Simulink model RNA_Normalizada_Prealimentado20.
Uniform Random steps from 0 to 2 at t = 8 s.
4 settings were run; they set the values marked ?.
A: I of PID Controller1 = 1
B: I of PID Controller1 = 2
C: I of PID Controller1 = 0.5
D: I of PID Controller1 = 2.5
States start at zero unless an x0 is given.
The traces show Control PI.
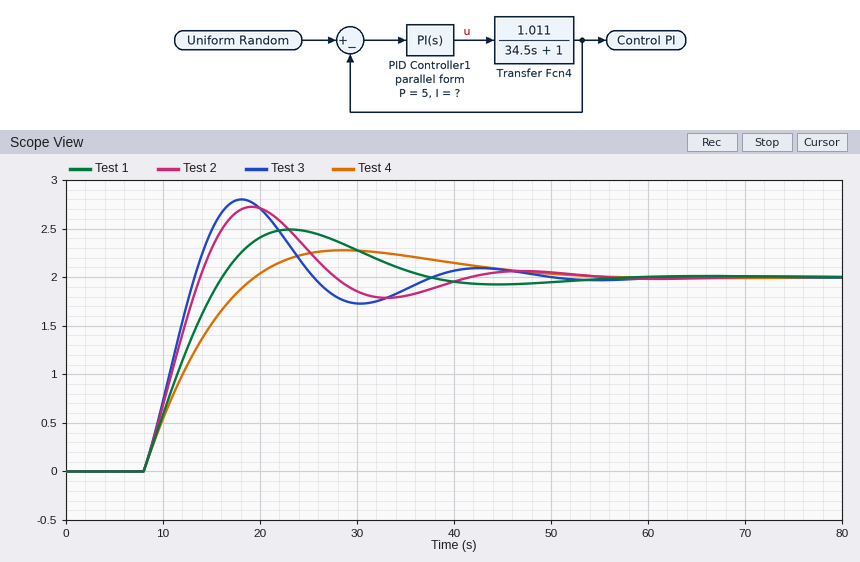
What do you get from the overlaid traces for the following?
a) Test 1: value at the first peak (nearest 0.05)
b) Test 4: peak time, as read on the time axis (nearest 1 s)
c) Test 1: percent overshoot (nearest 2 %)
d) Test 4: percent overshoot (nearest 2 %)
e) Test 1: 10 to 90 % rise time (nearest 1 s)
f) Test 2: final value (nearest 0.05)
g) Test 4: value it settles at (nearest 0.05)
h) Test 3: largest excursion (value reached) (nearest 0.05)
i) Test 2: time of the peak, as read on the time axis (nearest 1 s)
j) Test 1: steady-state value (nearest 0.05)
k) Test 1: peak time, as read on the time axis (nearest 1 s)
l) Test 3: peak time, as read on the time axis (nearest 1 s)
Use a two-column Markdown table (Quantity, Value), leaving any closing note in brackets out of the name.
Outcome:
| Quantity | Value |
|---|---|
| Test 1: value at the first peak | 2.50 |
| Test 4: peak time, as read on the time axis | 29 s |
| Test 1: percent overshoot | 24 % |
| Test 4: percent overshoot | 14 % |
| Test 1: 10 to 90 % rise time | 6 s |
| Test 2: final value | 2.00 |
| Test 4: value it settles at | 2.00 |
| Test 3: largest excursion (value reached) | 2.80 |
| Test 2: time of the peak, as read on the time axis | 19 s |
| Test 1: steady-state value | 2.00 |
| Test 1: peak time, as read on the time axis | 23 s |
| Test 3: peak time, as read on the time axis | 18 s |
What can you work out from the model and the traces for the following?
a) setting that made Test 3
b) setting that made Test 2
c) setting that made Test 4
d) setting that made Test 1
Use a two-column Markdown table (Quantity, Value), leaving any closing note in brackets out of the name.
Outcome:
| Quantity | Value |
|---|---|
| setting that made Test 3 | D |
| setting that made Test 2 | B |
| setting that made Test 4 | C |
| setting that made Test 1 | A |
